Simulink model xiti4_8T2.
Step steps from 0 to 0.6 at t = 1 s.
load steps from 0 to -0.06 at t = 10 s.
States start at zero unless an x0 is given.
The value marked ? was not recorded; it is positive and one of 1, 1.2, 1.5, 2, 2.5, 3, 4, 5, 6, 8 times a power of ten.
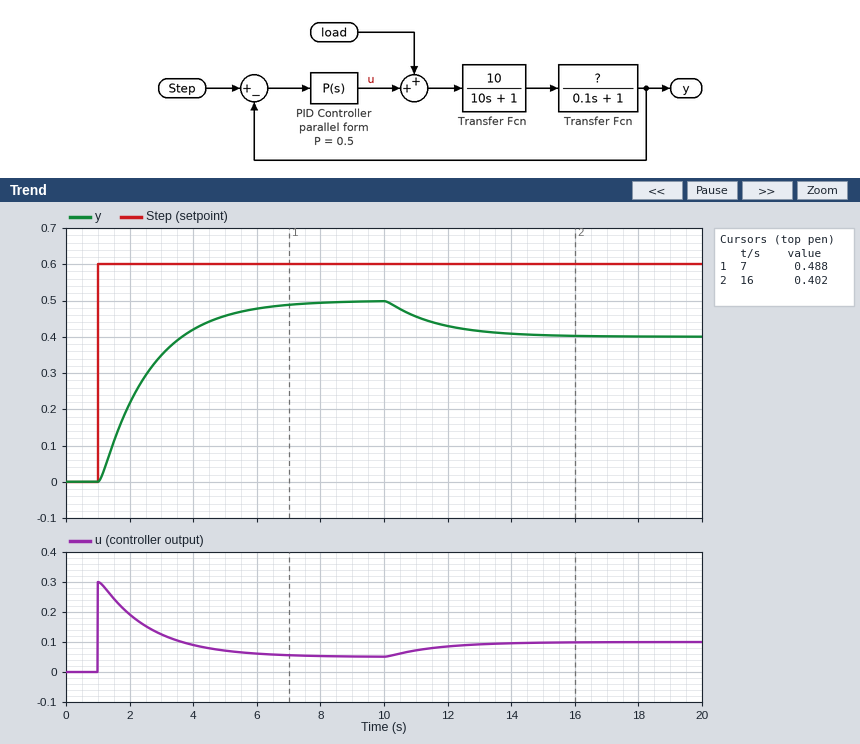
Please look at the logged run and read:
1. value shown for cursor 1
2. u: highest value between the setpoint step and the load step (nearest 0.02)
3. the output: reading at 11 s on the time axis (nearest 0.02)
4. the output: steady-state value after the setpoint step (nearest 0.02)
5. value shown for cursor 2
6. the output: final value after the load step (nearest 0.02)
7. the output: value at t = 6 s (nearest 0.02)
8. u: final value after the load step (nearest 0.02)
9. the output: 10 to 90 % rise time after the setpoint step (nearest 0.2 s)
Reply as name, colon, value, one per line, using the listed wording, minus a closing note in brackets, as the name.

value shown for cursor 1: 0.488
u: highest value between the setpoint step and the load step: 0.30
the output: reading at 11 s on the time axis: 0.46
the output: steady-state value after the setpoint step: 0.50
value shown for cursor 2: 0.402
the output: final value after the load step: 0.40
the output: value at t = 6 s: 0.48
u: final value after the load step: 0.10
the output: 10 to 90 % rise time after the setpoint step: 3.4 s
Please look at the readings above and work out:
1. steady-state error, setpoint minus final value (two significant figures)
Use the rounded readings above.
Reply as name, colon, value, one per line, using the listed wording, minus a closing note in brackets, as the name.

steady-state error, setpoint minus final value: 0.10
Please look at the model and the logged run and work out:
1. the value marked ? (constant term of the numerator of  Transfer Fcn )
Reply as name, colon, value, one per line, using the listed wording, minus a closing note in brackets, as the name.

the value marked ?: 1
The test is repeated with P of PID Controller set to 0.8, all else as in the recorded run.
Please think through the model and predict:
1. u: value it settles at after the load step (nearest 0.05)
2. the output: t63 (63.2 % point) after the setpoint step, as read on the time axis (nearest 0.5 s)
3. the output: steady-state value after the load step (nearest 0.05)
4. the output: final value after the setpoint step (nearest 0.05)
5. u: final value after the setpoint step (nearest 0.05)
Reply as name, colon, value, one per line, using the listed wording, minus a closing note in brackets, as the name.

u: value it settles at after the load step: 0.10
the output: t63 (63.2 % point) after the setpoint step, as read on the time axis: 2.0 s
the output: steady-state value after the load step: 0.45
the output: final value after the setpoint step: 0.55
u: final value after the setpoint step: 0.05
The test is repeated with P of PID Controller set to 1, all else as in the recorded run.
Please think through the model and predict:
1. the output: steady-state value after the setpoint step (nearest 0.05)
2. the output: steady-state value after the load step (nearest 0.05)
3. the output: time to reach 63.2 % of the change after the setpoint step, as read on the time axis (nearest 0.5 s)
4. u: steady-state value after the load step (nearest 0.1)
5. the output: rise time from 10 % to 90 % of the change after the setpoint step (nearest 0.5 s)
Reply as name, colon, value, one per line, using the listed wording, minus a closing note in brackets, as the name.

the output: steady-state value after the setpoint step: 0.55
the output: steady-state value after the load step: 0.50
the output: time to reach 63.2 % of the change after the setpoint step, as read on the time axis: 2.0 s
u: steady-state value after the load step: 0.1
the output: rise time from 10 % to 90 % of the change after the setpoint step: 2.0 s
